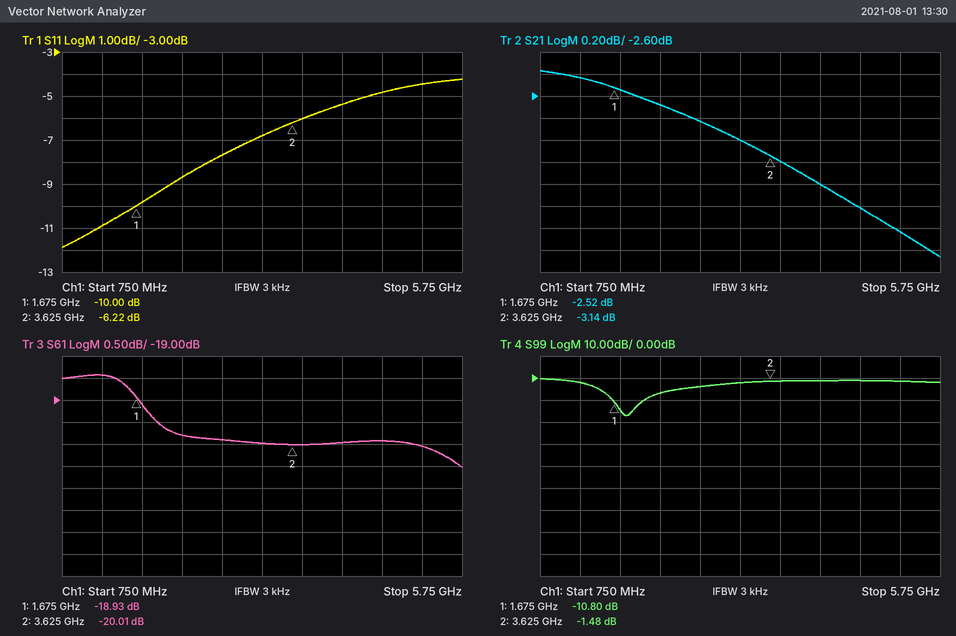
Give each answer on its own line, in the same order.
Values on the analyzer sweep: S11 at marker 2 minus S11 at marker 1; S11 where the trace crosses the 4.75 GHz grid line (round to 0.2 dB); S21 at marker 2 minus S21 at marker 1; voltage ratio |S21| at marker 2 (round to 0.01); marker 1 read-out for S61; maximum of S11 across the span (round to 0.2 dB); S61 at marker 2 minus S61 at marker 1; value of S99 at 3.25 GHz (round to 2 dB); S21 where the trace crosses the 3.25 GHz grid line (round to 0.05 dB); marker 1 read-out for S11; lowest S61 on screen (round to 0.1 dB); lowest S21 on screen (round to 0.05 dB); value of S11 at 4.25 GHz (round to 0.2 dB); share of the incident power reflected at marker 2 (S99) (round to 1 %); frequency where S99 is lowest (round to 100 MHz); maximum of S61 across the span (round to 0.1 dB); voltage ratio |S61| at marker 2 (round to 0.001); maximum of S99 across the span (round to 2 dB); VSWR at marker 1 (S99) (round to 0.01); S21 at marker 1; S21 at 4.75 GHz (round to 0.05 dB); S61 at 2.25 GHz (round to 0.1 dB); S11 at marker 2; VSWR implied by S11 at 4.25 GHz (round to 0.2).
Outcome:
3.78 dB
-4.8 dB
-0.62 dB
0.70
-18.93 dB
-4.2 dB
-1.08 dB
-2 dB
-3.00 dB
-10.00 dB
-20.5 dB
-4.05 dB
-5.4 dB
71 %
1.8 GHz
-18.4 dB
0.100
0 dB
1.81
-2.52 dB
-3.60 dB
-19.8 dB
-6.22 dB
3.4
